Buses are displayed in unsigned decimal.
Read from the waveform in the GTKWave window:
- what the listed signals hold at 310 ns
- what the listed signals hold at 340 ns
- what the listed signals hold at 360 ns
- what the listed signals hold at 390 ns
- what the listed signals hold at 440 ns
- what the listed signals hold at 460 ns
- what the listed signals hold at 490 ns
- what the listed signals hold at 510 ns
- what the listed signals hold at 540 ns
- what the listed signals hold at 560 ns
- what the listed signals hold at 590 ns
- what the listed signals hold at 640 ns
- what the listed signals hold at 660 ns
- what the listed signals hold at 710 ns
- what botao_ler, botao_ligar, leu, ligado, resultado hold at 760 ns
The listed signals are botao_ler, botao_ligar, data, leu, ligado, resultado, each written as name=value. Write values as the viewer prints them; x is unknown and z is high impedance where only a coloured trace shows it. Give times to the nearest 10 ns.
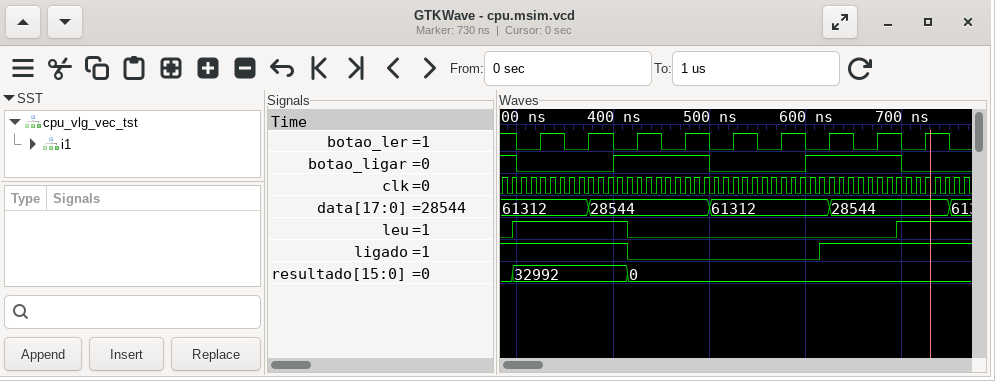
botao_ler=0, botao_ligar=0, data=61312, leu=1, ligado=1, resultado=32992
botao_ler=1, botao_ligar=0, data=61312, leu=1, ligado=1, resultado=32992
botao_ler=0, botao_ligar=0, data=61312, leu=1, ligado=1, resultado=32992
botao_ler=1, botao_ligar=0, data=28544, leu=1, ligado=1, resultado=32992
botao_ler=1, botao_ligar=1, data=28544, leu=0, ligado=0, resultado=0
botao_ler=0, botao_ligar=1, data=28544, leu=0, ligado=0, resultado=0
botao_ler=1, botao_ligar=1, data=28544, leu=0, ligado=0, resultado=0
botao_ler=0, botao_ligar=0, data=61312, leu=0, ligado=0, resultado=0
botao_ler=1, botao_ligar=0, data=61312, leu=0, ligado=0, resultado=0
botao_ler=0, botao_ligar=0, data=61312, leu=0, ligado=0, resultado=0
botao_ler=1, botao_ligar=0, data=61312, leu=0, ligado=0, resultado=0
botao_ler=1, botao_ligar=1, data=28544, leu=0, ligado=1, resultado=0
botao_ler=0, botao_ligar=1, data=28544, leu=0, ligado=1, resultado=0
botao_ler=0, botao_ligar=0, data=28544, leu=1, ligado=1, resultado=0
botao_ler=0, botao_ligar=0, leu=1, ligado=1, resultado=0
